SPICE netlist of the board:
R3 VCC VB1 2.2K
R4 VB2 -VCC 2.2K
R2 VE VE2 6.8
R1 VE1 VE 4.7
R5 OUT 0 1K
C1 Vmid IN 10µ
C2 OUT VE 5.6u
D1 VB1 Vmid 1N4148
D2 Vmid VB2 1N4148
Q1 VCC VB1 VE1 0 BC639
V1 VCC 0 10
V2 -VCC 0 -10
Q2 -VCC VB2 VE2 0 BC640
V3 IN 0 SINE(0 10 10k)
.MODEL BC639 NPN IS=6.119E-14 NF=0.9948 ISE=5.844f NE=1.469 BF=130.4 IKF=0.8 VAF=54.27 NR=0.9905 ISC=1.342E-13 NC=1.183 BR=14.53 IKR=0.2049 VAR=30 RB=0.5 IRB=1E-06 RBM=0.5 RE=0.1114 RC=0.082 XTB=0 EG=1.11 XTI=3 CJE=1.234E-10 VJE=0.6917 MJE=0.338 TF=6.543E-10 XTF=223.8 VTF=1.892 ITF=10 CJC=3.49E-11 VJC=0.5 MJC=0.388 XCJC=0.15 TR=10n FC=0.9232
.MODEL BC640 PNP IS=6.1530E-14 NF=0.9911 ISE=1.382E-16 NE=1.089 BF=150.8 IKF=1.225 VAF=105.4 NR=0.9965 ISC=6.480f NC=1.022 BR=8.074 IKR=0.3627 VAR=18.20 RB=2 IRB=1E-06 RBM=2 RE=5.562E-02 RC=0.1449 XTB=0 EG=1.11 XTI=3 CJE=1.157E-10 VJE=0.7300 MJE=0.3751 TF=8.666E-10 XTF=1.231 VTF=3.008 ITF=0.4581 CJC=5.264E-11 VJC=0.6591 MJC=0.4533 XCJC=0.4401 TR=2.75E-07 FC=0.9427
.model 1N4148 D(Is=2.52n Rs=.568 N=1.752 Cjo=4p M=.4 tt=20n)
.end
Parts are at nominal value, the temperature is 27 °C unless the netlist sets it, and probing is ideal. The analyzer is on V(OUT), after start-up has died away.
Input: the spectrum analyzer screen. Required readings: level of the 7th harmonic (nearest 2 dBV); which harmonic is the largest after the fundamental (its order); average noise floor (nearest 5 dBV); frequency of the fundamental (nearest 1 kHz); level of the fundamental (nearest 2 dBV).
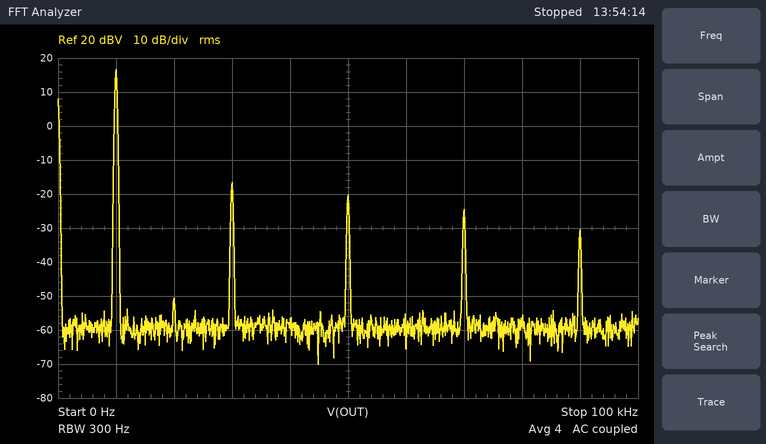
-24 dBV
3
-60 dBV
10 kHz
16 dBV
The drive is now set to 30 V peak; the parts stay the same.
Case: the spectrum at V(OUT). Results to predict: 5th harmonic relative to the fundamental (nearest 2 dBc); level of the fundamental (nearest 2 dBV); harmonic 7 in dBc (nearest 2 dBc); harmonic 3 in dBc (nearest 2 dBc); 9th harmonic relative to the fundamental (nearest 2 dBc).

-18 dBc
18 dBV
-26 dBc
-10 dBc
-38 dBc
